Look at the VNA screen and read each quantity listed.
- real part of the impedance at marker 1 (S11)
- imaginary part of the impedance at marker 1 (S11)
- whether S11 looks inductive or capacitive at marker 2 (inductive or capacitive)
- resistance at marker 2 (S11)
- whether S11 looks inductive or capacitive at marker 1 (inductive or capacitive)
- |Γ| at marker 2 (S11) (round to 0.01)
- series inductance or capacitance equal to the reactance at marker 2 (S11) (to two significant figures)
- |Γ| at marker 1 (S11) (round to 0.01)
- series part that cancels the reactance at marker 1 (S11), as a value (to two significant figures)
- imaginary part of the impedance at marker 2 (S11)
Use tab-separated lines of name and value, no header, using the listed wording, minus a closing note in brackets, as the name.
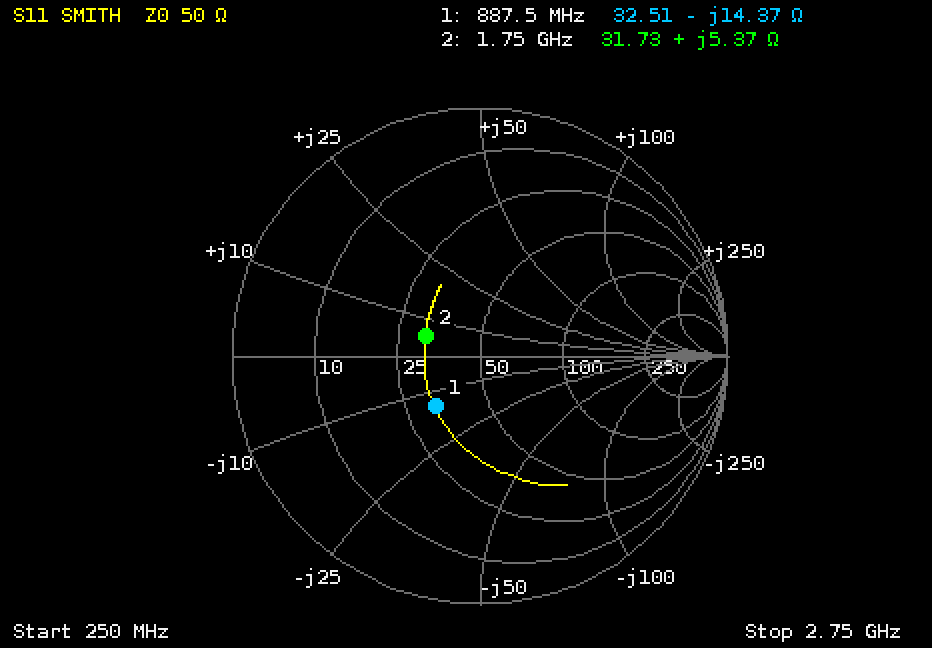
real part of the impedance at marker 1	32.51 Ω
imaginary part of the impedance at marker 1	-14.37 Ω
whether S11 looks inductive or capacitive at marker 2	inductive
resistance at marker 2	31.73 Ω
whether S11 looks inductive or capacitive at marker 1	capacitive
|Γ| at marker 2 (S11)	0.23
series inductance or capacitance equal to the reactance at marker 2 (S11)	490 pH
|Γ| at marker 1 (S11)	0.27
series part that cancels the reactance at marker 1 (S11), as a value	2.6 nH
imaginary part of the impedance at marker 2	+5.37 Ω
